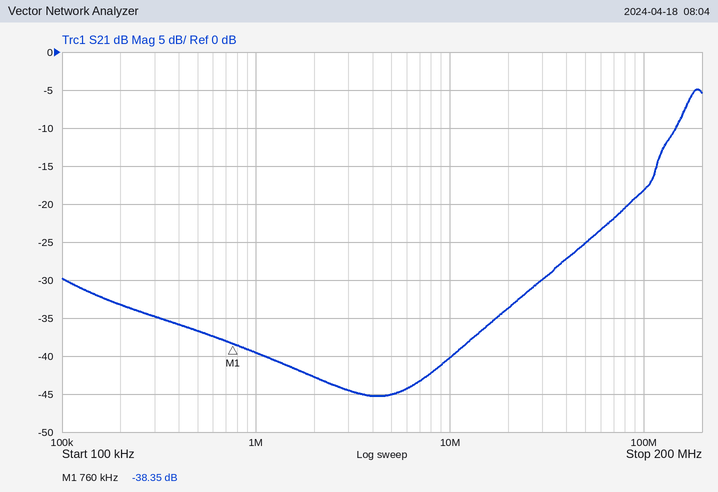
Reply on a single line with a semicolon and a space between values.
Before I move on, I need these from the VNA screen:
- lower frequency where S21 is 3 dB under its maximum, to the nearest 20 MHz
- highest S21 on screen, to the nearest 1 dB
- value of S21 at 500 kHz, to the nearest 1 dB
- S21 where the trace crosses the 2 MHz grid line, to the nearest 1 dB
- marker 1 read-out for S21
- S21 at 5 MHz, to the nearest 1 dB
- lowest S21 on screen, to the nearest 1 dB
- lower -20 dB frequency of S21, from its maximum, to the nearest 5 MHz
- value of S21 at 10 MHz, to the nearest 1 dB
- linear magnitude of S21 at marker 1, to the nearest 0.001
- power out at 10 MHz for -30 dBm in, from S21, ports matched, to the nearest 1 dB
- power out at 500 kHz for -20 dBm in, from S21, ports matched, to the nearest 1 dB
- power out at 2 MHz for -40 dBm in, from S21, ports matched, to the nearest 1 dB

160 MHz; -5 dB; -37 dB; -43 dB; -38.35 dB; -45 dB; -45 dB; 50 MHz; -40 dB; 0.012; -70 dBm; -57 dBm; -83 dBm
